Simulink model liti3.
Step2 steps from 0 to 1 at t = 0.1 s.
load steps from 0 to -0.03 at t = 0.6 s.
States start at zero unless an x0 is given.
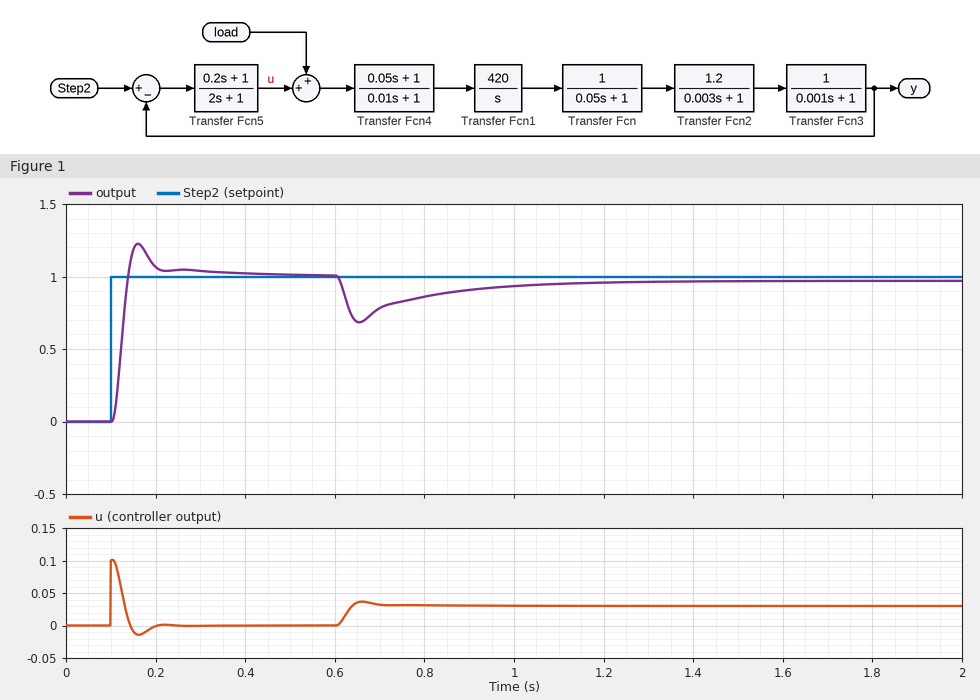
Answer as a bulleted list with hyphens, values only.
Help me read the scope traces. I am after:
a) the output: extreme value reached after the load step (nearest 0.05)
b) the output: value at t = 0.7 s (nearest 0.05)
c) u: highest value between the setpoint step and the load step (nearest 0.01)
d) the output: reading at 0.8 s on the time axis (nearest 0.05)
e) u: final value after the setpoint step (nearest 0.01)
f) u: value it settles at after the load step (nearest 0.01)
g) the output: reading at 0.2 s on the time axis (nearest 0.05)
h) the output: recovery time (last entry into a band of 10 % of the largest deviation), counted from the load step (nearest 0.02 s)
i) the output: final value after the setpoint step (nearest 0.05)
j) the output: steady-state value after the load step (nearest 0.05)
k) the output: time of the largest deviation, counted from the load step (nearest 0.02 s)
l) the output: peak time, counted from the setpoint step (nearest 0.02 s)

- 0.70
- 0.80
- 0.10
- 0.85
- 0.00
- 0.03
- 1.05
- 0.42 s
- 1.00
- 0.95
- 0.06 s
- 0.06 s
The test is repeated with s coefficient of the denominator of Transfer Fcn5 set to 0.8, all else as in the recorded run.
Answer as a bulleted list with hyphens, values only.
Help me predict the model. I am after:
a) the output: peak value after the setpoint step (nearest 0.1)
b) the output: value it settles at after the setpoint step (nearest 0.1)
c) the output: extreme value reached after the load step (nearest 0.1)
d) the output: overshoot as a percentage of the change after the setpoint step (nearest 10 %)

- 1.5
- 1.0
- 0.8
- 50 %
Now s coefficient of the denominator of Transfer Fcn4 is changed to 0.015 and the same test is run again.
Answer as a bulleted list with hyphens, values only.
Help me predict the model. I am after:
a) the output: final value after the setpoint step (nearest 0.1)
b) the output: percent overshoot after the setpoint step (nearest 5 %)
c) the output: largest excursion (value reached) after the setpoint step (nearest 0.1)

- 1.0
- 30 %
- 1.3
